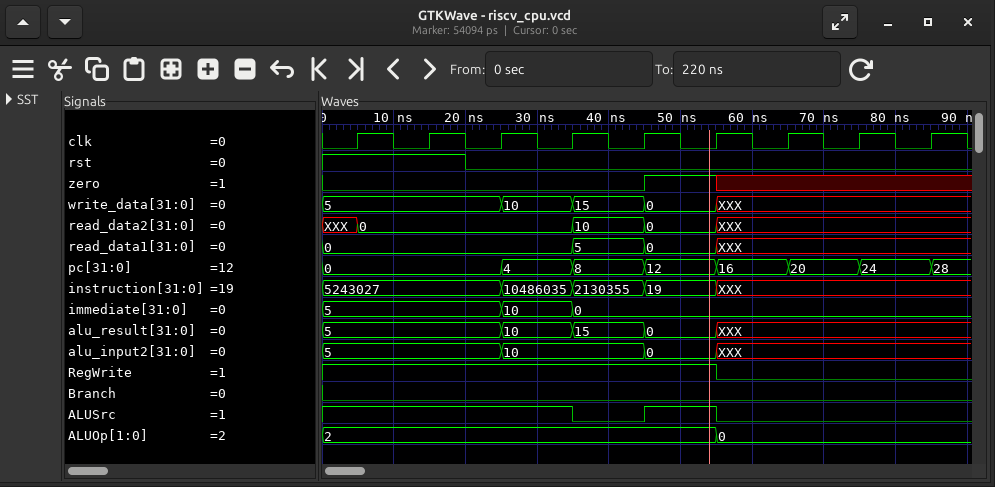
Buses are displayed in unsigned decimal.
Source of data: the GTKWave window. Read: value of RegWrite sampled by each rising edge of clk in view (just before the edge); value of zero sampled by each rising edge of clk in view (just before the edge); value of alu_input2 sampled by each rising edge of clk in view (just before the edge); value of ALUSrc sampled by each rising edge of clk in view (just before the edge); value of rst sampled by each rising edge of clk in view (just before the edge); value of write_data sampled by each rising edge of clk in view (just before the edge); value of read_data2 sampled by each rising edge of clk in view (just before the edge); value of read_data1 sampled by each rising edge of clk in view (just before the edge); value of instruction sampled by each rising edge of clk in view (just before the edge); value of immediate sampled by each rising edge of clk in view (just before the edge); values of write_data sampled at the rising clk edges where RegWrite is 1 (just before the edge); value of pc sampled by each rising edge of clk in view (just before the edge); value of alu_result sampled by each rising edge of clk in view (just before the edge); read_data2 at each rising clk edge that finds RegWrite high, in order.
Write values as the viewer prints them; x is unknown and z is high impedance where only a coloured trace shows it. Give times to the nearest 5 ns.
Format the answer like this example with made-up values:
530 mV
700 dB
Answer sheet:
1 1 1 1 1 1 0 0 0
0 0 0 0 0 1 x x x
5, 5, 5, 10, 10, 0, XXX, XXX, XXX
1 1 1 1 0 1 0 0 0
1 1 0 0 0 0 0 0 0
5, 5, 5, 10, 15, 0, XXX, XXX, XXX
XXX, 0, 0, 0, 10, 0, XXX, XXX, XXX
0, 0, 0, 0, 5, 0, XXX, XXX, XXX
5243027, 5243027, 5243027, 10486035, 2130355, 19, XXX, XXX, XXX
5, 5, 5, 10, 0, 0, 0, 0, 0
5, 5, 5, 10, 15, 0
0, 0, 0, 4, 8, 12, 16, 20, 24
5, 5, 5, 10, 15, 0, XXX, XXX, XXX
XXX, 0, 0, 0, 10, 0
